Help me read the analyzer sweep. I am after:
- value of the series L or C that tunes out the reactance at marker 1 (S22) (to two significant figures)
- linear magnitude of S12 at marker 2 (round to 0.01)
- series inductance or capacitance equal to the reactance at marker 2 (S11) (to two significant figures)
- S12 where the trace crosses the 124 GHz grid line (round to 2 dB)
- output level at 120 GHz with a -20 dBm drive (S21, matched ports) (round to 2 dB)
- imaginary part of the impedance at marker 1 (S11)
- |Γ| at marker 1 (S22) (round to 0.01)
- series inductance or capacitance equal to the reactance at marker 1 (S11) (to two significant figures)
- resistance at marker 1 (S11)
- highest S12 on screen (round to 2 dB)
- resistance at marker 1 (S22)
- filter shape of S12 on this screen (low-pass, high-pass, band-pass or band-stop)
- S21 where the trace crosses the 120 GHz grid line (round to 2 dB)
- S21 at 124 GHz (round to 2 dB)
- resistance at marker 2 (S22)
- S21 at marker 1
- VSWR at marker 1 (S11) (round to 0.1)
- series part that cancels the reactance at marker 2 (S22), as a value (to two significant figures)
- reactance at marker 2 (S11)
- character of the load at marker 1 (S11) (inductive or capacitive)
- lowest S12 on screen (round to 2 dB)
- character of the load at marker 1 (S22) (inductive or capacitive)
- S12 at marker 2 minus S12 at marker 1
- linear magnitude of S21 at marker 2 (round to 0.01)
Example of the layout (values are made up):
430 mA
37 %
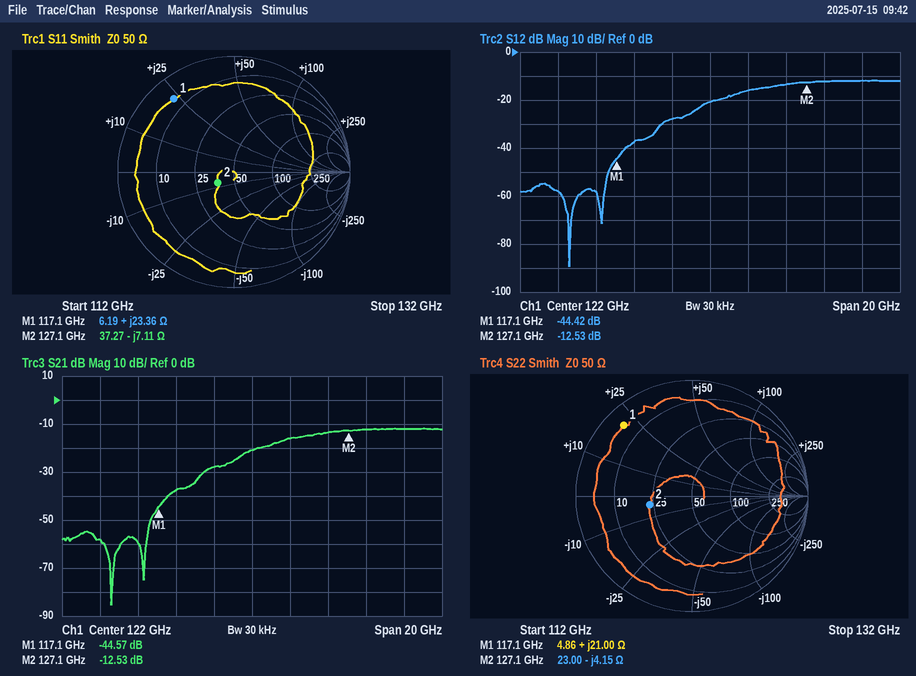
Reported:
65 fF
0.24
180 fF
-16 dB
-48 dBm
+23.36 Ω
0.85
32 pH
6.19 Ω
-12 dB
4.86 Ω
high-pass
-28 dB
-16 dB
23.00 Ω
-44.57 dB
9.9
5.2 pH
-7.11 Ω
inductive
-90 dB
inductive
31.89 dB
0.24
